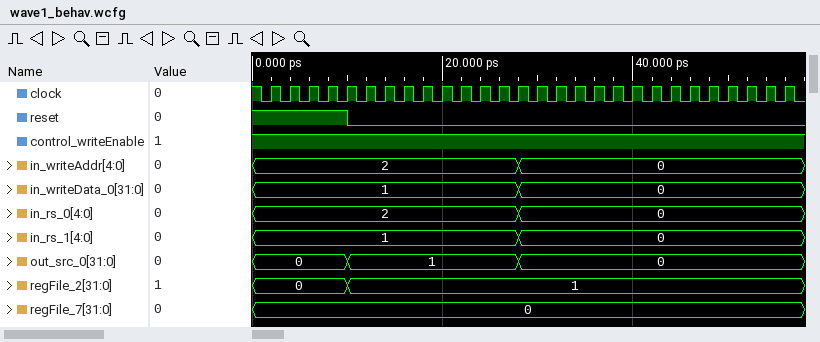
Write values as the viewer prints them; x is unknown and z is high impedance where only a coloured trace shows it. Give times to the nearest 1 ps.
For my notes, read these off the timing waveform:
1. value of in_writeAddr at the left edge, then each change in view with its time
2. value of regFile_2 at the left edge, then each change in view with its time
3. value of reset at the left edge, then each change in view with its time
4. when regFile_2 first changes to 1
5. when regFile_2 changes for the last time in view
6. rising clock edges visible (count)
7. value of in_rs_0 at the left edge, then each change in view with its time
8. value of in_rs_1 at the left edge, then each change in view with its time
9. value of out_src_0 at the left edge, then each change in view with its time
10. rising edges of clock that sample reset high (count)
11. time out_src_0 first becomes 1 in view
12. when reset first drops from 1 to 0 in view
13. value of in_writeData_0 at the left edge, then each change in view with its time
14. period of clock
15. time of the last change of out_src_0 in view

2, 0 at 28 ps
0, 1 at 10 ps
1, 0 at 10 ps
10 ps
10 ps
28
2, 0 at 28 ps
1, 0 at 28 ps
0, 1 at 10 ps, 0 at 28 ps
5
10 ps
10 ps
1, 0 at 28 ps
2 ps
28 ps
